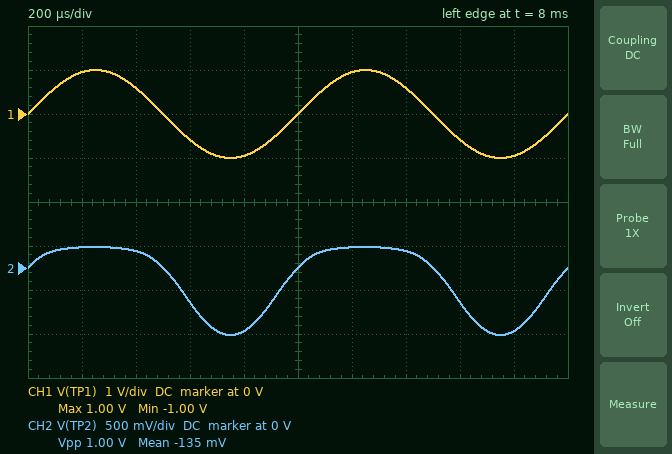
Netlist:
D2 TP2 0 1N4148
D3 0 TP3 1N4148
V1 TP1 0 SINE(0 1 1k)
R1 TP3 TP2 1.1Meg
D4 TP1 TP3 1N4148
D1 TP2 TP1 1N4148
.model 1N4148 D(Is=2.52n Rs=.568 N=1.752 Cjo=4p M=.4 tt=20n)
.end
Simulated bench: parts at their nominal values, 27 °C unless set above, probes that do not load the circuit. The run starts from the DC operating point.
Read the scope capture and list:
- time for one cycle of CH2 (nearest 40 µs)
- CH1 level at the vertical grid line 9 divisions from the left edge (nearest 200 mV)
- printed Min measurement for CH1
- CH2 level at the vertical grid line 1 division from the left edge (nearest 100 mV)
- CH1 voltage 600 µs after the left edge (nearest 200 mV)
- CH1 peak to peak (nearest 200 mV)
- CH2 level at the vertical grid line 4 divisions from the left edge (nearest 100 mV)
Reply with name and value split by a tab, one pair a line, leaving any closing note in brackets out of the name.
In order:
time for one cycle of CH2	1.00 ms
CH1 level at the vertical grid line 9 divisions from the left edge	-1.0 V
printed Min measurement for CH1	-1.00 V
CH2 level at the vertical grid line 1 division from the left edge	200 mV
CH1 voltage 600 µs after the left edge	-600 mV
CH1 peak to peak	2.0 V
CH2 level at the vertical grid line 4 divisions from the left edge	-700 mV
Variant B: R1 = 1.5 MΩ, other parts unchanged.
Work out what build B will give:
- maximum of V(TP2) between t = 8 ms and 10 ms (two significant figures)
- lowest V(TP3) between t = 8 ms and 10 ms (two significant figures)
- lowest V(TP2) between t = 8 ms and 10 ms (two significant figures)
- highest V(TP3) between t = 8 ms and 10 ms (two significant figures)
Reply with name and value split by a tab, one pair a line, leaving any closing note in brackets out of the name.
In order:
maximum of V(TP2) between t = 8 ms and 10 ms	230 mV
lowest V(TP3) between t = 8 ms and 10 ms	-230 mV
lowest V(TP2) between t = 8 ms and 10 ms	-770 mV
highest V(TP3) between t = 8 ms and 10 ms	770 mV
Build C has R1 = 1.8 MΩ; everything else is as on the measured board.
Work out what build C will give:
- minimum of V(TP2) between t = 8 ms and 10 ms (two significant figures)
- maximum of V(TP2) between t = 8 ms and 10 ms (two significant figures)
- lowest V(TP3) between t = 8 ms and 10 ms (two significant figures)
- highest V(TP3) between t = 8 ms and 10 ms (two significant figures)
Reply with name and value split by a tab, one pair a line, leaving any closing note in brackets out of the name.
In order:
minimum of V(TP2) between t = 8 ms and 10 ms	-780 mV
maximum of V(TP2) between t = 8 ms and 10 ms	220 mV
lowest V(TP3) between t = 8 ms and 10 ms	-220 mV
highest V(TP3) between t = 8 ms and 10 ms	780 mV
